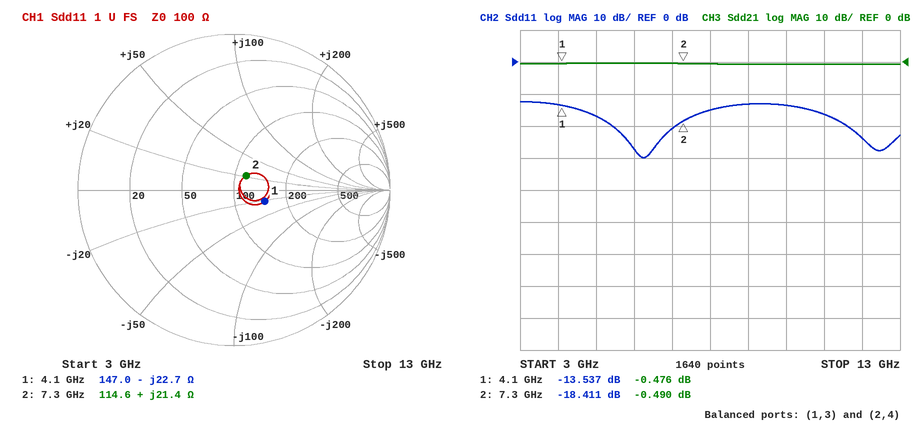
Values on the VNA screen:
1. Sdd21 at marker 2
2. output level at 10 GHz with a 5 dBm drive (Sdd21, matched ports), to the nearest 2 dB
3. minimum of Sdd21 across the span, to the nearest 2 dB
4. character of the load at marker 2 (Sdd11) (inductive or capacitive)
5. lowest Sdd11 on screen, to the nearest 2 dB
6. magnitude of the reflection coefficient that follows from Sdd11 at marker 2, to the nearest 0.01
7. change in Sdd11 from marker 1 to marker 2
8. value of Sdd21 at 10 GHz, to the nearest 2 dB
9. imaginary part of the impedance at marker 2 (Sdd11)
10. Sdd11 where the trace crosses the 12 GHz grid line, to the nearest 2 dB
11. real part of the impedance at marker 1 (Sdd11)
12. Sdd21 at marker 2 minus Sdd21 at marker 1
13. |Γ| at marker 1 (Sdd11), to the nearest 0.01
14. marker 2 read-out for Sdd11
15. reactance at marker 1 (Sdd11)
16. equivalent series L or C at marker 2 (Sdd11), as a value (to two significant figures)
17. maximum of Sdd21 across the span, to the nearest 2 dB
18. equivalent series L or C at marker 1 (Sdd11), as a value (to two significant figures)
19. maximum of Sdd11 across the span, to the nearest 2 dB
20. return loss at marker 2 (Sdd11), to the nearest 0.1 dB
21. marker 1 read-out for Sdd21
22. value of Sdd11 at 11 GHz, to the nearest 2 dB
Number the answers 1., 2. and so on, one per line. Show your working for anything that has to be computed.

1. -0.490 dB
2. 5 dBm + (0 dB) = 4 dBm
3. 0 dB
4. inductive
5. -30 dB
6. 10^(-18.411/20) ≈ 0.12
7. -18.411 − (-13.537) = -4.874 dB
8. 0 dB
9. +21.4 Ω
10. -24 dB
11. 147.0 Ω
12. -0.49 − (-0.476) = -0.014 dB
13. 0.21
14. -18.411 dB
15. -22.7 Ω
16. L = 21.4 Ω/(2π × 7.3 GHz) ≈ 467 pH, so 470 pH to two significant figures
17. 0 dB
18. C = 1/(2π × 4.1 GHz × 22.7 Ω) ≈ 1.7 pF
19. -12 dB
20. 18.4 dB
21. -0.476 dB
22. -16 dB
